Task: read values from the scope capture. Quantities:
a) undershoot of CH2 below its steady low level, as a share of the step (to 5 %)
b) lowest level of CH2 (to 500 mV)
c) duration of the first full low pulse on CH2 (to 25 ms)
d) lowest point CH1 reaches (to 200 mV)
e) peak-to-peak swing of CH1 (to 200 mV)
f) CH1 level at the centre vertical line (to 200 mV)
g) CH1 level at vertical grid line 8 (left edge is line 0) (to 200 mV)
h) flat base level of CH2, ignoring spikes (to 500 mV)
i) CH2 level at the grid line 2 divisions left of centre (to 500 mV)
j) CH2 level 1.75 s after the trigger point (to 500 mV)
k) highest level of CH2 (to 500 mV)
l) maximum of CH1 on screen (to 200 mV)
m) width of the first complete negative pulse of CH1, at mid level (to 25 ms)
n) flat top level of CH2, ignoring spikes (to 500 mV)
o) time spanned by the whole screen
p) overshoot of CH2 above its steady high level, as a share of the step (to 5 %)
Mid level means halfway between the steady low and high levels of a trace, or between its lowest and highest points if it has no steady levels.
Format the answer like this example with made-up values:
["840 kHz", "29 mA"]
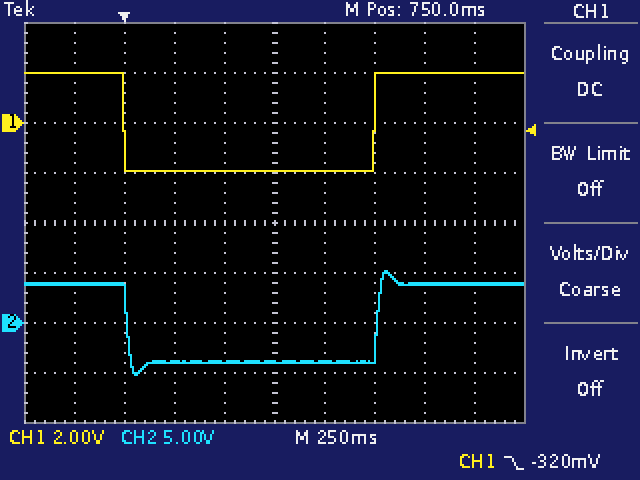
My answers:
["15 %", "-5.0 V", "1.250 s", "-2.0 V", "4.0 V", "-2.0 V", "2.0 V", "-4.0 V", "-4.0 V", "4.0 V", "5.0 V", "2.0 V", "1.250 s", "4.0 V", "2.5 s", "15 %"]
